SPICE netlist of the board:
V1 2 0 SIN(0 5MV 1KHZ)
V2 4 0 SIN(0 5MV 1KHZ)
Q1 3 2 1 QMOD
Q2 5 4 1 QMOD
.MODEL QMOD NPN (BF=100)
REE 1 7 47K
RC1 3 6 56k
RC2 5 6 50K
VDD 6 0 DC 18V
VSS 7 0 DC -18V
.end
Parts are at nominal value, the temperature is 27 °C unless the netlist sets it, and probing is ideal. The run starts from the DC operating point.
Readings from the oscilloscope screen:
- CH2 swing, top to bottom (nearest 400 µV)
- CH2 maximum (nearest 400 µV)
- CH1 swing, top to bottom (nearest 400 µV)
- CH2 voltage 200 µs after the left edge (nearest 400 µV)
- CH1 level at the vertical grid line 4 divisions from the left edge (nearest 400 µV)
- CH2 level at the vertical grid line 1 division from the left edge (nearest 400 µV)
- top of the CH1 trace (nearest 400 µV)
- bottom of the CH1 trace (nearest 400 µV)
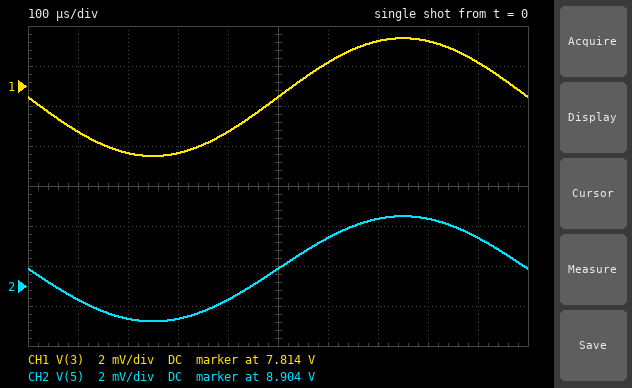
5.2 mV
8.9076 V
6.0 mV
8.9024 V
7.8116 V
8.9032 V
7.8164 V
7.8104 V
